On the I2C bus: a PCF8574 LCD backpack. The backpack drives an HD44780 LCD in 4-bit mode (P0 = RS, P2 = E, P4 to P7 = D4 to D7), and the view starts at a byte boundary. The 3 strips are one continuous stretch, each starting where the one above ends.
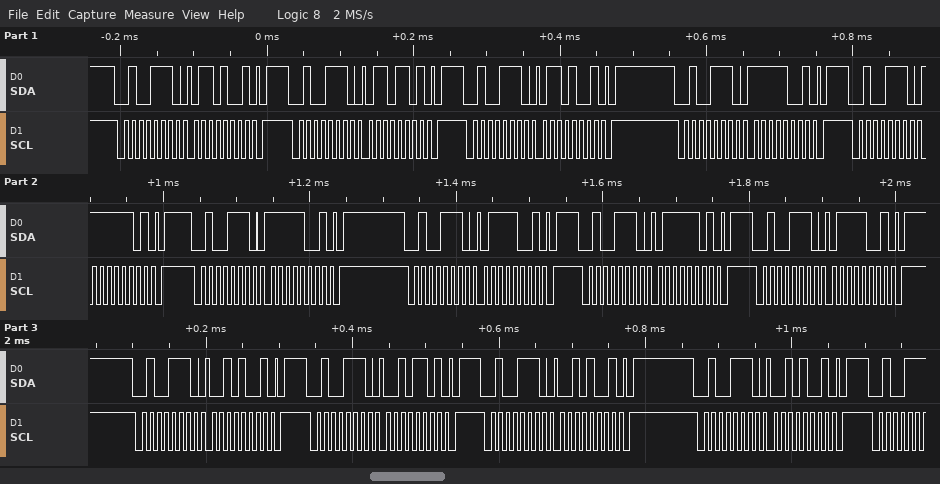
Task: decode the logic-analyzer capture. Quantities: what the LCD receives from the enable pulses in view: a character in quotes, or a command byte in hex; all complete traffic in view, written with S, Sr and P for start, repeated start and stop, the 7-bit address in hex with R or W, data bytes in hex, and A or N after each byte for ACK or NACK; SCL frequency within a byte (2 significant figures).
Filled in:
'o' 'r'
S 27W A 69 A P S 27W A 6D A P S 27W A 69 A P S 27W A F9 A P S 27W A FD A P S 27W A F9 A P S 27W A 79 A P S 27W A 7D A P S 27W A 79 A P S 27W A 29 A P S 27W A 2D A P S 27W A 29 A P S 27W A 29 A P
100 kHz
